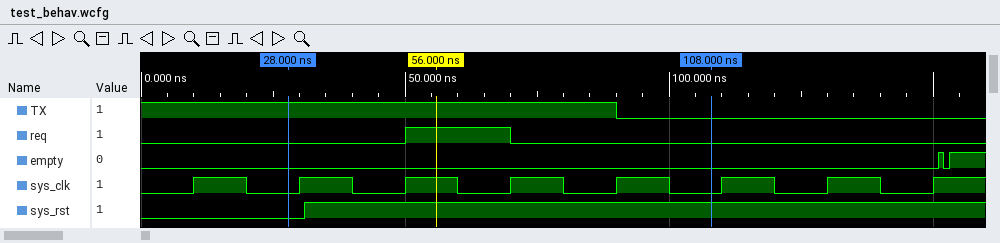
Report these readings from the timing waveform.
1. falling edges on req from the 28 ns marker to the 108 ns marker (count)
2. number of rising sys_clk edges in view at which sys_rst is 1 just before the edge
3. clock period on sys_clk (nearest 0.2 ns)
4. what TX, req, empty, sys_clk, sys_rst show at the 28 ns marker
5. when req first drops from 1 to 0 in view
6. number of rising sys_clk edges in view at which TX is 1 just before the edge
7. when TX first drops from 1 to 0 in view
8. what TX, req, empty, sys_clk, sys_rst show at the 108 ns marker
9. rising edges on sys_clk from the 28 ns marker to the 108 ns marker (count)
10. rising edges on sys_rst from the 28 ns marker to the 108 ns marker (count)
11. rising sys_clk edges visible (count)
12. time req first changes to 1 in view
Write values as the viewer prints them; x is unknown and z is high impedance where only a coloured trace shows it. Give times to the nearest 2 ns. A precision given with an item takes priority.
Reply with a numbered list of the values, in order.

1. 1
2. 6
3. 20 ns
4. TX=1, req=0, empty=0, sys_clk=0, sys_rst=0
5. 70 ns
6. 5
7. 90 ns
8. TX=0, req=0, empty=0, sys_clk=0, sys_rst=1
9. 4
10. 1
11. 8
12. 50 ns
